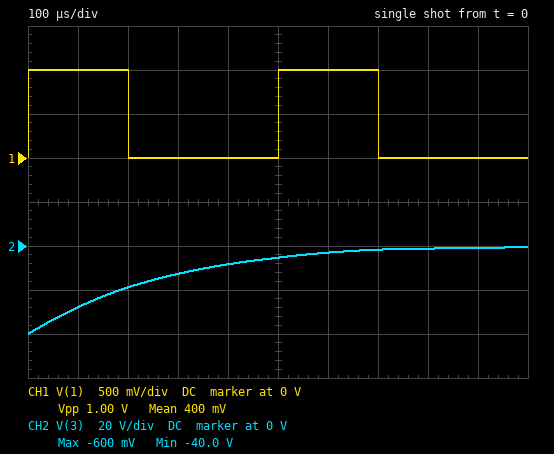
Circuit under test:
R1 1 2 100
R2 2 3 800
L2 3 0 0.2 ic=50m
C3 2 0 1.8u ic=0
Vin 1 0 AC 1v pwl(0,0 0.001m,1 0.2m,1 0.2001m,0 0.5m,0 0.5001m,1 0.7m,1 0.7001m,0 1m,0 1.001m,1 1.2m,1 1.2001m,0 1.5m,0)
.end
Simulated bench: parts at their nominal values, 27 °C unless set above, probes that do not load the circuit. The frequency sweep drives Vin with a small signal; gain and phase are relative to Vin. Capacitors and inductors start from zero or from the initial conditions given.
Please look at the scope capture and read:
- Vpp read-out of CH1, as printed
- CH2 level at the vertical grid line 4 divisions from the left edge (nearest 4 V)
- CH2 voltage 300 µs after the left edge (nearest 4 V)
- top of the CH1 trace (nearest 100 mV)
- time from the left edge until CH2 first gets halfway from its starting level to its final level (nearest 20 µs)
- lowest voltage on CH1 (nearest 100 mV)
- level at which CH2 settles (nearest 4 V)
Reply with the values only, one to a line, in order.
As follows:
1.00 V
-8 V
-12 V
1.0 V
180 µs
0 V
0 V
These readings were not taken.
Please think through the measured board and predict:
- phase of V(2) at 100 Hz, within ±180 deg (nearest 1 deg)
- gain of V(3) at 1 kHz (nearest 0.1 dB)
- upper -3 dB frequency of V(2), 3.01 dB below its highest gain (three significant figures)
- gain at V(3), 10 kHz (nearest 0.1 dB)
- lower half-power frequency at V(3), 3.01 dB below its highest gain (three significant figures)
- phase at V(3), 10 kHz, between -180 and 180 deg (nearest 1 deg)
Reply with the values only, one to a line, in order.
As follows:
-5 deg
-5.0 dB
1.12 kHz
-21.1 dB
340 Hz
-81 deg
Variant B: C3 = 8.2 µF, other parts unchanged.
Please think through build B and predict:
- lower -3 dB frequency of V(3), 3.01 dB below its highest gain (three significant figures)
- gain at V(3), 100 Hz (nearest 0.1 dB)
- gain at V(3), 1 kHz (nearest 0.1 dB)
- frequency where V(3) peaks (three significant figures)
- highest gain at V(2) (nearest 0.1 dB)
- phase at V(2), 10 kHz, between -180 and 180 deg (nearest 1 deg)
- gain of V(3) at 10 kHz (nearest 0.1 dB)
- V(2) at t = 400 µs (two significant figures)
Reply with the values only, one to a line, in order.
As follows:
143 Hz
-18.0 dB
-15.8 dB
373 Hz
-1.0 dB
-89 deg
-34.3 dB
-720 mV
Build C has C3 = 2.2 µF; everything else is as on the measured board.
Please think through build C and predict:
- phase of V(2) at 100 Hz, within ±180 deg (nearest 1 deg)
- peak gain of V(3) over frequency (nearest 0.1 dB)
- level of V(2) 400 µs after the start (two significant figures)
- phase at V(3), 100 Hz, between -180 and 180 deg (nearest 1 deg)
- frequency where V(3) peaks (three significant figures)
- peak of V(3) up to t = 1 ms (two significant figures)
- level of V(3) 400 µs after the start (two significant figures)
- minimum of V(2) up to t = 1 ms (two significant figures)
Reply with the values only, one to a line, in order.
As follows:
-6 deg
-5.5 dB
-1.3 V
75 deg
720 Hz
-540 mV
-8.4 V
-1.5 V
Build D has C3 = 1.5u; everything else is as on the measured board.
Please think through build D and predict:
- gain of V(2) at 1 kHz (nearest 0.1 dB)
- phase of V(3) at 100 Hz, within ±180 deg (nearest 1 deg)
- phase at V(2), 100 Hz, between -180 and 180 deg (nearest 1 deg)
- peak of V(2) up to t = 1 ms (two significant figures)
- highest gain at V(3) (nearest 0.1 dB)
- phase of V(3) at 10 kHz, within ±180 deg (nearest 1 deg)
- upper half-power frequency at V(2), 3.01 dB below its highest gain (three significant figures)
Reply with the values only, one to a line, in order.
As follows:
-2.7 dB
77 deg
-4 deg
240 mV
-4.1 dB
-80 deg
1.34 kHz
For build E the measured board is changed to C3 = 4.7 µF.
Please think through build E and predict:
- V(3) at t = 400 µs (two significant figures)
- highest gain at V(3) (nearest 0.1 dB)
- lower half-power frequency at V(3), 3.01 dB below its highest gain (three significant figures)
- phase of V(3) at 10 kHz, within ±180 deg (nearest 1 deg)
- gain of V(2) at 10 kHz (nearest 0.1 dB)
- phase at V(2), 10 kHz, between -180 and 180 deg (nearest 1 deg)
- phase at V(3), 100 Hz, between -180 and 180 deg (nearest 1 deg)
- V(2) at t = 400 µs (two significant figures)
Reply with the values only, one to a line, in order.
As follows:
-8.4 V
-9.2 dB
205 Hz
-84 deg
-29.4 dB
-88 deg
67 deg
-1.0 V
